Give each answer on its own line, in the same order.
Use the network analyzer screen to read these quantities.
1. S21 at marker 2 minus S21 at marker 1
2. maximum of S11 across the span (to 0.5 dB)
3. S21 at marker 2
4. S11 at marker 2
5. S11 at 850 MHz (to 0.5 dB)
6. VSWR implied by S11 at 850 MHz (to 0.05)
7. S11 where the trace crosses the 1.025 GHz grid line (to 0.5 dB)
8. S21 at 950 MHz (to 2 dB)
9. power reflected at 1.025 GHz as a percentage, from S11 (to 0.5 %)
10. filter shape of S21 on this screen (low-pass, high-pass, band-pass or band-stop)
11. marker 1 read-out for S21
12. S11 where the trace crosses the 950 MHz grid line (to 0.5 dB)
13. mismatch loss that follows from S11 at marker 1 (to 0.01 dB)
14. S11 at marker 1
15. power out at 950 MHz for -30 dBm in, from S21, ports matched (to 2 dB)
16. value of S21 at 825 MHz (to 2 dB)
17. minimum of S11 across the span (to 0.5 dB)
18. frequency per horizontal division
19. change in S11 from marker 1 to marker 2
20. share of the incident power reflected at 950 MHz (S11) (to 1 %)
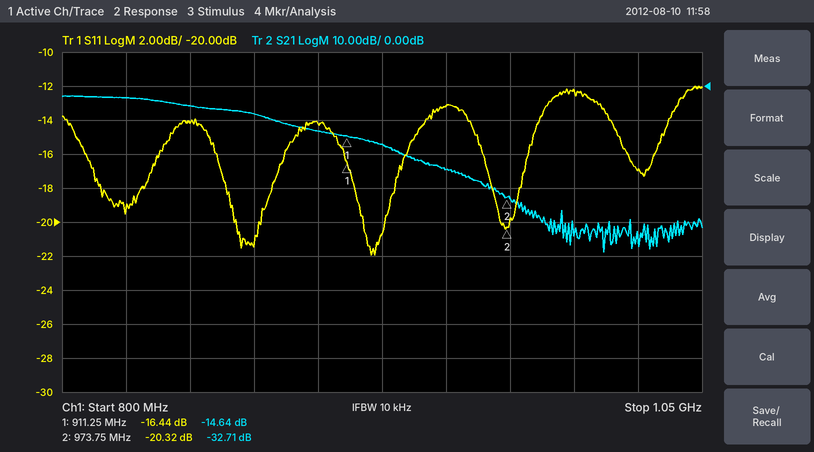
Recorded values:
-18.07 dB
-12.0 dB
-32.71 dB
-20.32 dB
-14.0 dB
1.50
-17.0 dB
-24 dB
2.0 %
low-pass
-14.64 dB
-13.0 dB
0.10 dB
-16.44 dB
-54 dBm
-4 dB
-22.0 dB
25 MHz
-3.88 dB
5 %
